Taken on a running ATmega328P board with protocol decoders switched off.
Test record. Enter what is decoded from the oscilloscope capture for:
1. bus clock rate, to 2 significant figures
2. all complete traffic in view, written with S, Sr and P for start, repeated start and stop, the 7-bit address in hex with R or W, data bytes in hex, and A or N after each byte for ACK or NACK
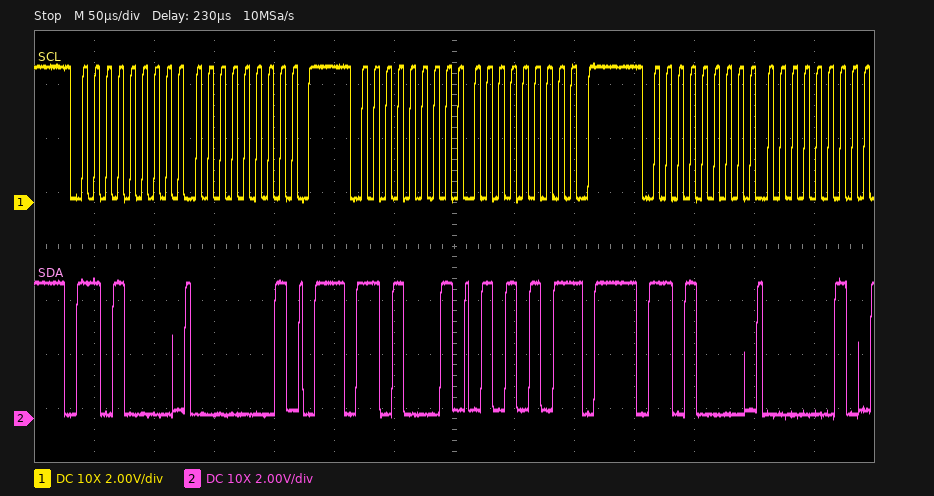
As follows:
100 kHz
S 68W A 01 A P S 68R A 55 N P S 68W A 02 A
